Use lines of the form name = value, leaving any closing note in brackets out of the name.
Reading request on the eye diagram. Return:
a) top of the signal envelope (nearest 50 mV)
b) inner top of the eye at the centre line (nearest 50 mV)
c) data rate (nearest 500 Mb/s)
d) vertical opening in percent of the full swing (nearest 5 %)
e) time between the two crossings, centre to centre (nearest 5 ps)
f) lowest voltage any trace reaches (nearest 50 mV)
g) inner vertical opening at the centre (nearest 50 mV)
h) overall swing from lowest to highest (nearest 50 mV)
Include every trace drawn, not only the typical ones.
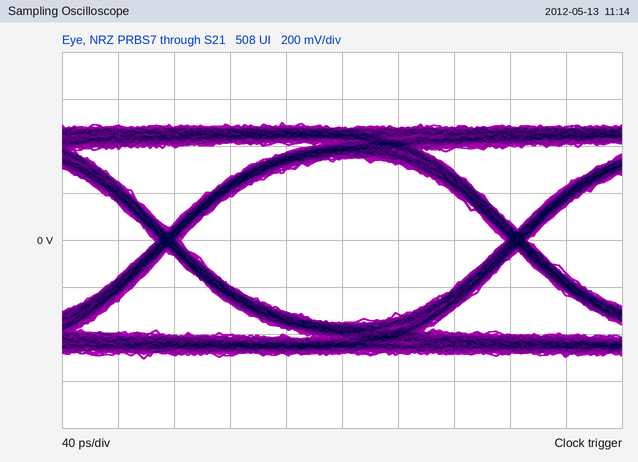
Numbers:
top of the signal envelope = 500 mV
inner top of the eye at the centre line = 350 mV
data rate = 4.0 Gb/s
vertical opening in percent of the full swing = 70 %
time between the two crossings, centre to centre = 250 ps
lowest voltage any trace reaches = -500 mV
inner vertical opening at the centre = 700 mV
overall swing from lowest to highest = 1.00 V
